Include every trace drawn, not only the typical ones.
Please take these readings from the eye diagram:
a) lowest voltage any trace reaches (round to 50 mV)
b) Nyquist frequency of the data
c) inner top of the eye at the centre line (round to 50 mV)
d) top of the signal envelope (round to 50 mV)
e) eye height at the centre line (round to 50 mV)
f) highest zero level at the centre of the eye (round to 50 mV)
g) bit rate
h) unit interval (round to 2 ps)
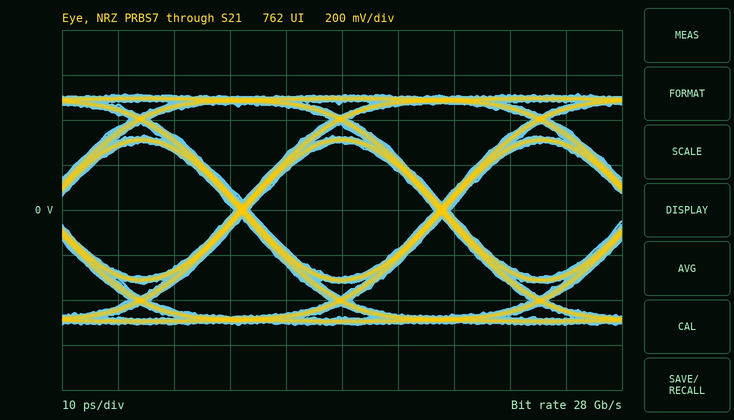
-500 mV
14 GHz
300 mV
500 mV
600 mV
-300 mV
28 Gb/s
36 ps
